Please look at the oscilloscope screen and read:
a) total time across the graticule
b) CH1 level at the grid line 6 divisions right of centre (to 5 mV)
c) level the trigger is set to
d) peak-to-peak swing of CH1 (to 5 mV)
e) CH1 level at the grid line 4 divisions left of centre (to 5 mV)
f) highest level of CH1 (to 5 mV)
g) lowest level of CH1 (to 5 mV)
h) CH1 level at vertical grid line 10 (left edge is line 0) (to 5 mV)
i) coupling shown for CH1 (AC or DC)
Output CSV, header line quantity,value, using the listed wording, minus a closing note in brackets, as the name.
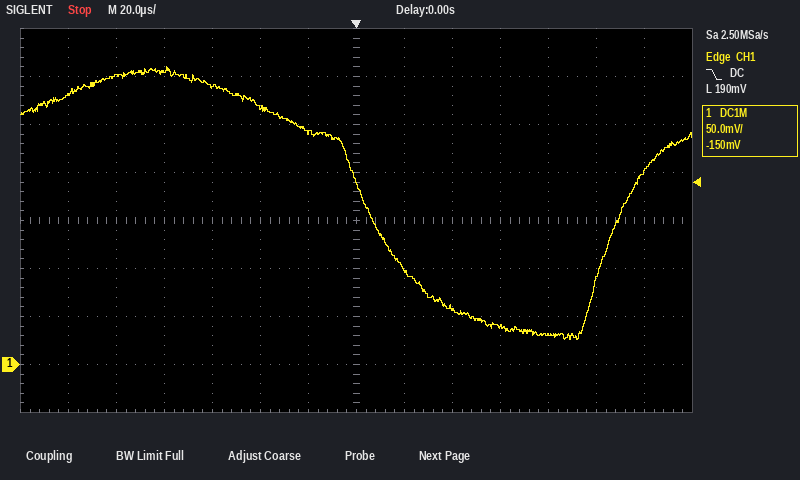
quantity,value
total time across the graticule,280 µs
CH1 level at the grid line 6 divisions right of centre,200 mV
level the trigger is set to,190 mV
peak-to-peak swing of CH1,285 mV
CH1 level at the grid line 4 divisions left of centre,305 mV
highest level of CH1,310 mV
lowest level of CH1,25 mV
CH1 level at vertical grid line 10 (left edge is line 0),40 mV
coupling shown for CH1,DC
